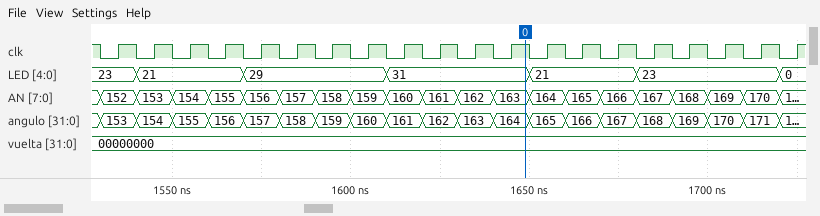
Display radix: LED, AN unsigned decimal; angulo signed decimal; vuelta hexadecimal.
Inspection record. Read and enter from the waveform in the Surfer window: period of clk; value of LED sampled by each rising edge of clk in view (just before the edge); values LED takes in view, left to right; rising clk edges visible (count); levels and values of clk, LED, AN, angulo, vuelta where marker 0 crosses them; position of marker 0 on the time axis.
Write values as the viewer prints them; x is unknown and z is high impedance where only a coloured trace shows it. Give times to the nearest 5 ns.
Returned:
10 ns
23, 21, 21, 21, 29, 29, 29, 29, 31, 31, 31, 31, 21, 21, 21, 23, 23, 23, 23, 0
23, 21, 29, 31, 21, 23, 0
20
clk=1, LED=31, AN=163, angulo=164, vuelta=00000000
1650 ns
